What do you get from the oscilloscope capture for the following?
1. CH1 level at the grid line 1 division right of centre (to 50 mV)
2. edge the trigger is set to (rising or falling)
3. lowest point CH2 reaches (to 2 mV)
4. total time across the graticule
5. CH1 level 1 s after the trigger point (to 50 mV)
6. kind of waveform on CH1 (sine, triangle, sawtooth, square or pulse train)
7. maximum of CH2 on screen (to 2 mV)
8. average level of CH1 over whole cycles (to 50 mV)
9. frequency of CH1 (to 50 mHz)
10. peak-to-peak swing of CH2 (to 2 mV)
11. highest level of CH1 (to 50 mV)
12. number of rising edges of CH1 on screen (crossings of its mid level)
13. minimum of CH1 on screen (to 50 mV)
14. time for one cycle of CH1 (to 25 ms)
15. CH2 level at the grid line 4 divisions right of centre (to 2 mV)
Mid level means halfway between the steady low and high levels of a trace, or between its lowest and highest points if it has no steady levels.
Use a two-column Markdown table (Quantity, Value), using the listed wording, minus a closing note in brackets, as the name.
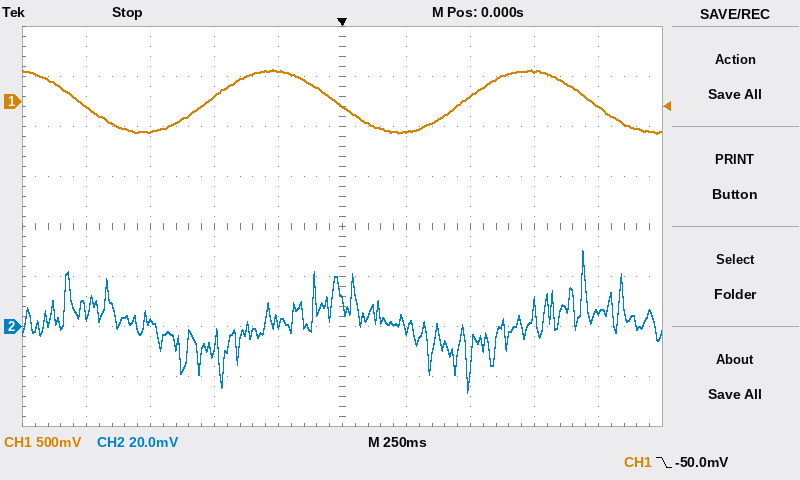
| Quantity | Value |
|---|---|
| CH1 level at the grid line 1 division right of centre | -300 mV |
| edge the trigger is set to | falling |
| lowest point CH2 reaches | -26 mV |
| total time across the graticule | 2.5 s |
| CH1 level 1 s after the trigger point | -50 mV |
| kind of waveform on CH1 | sine |
| maximum of CH2 on screen | 30 mV |
| average level of CH1 over whole cycles | 0 mV |
| frequency of CH1 | 1.00 Hz |
| peak-to-peak swing of CH2 | 56 mV |
| highest level of CH1 | 300 mV |
| number of rising edges of CH1 on screen | 2 |
| minimum of CH1 on screen | -300 mV |
| time for one cycle of CH1 | 1.000 s |
| CH2 level at the grid line 4 divisions right of centre | 6 mV |
